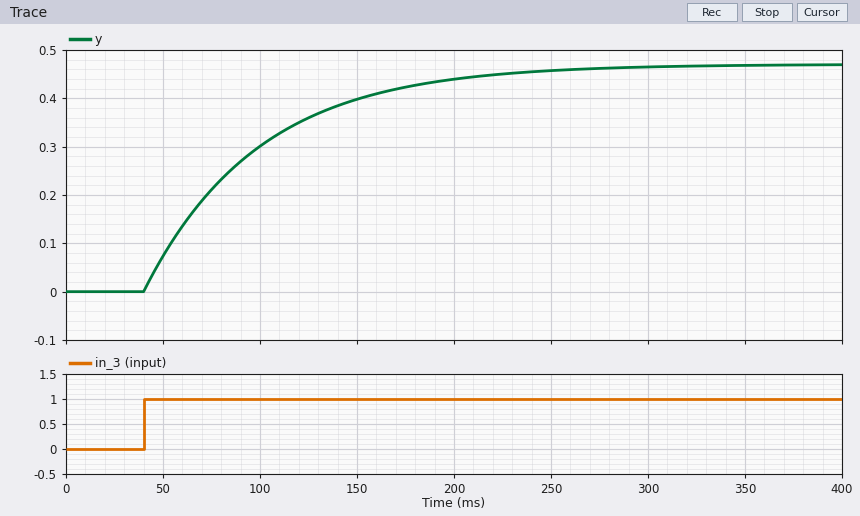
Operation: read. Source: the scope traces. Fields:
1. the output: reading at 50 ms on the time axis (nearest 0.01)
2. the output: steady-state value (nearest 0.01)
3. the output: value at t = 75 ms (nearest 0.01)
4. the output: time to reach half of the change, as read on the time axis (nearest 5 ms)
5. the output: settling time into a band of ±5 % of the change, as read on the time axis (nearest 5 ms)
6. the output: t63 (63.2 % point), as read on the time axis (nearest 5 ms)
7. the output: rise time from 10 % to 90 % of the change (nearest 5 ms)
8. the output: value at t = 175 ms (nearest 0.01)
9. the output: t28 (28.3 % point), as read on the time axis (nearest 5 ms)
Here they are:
0.07
0.47
0.21
80 ms
215 ms
100 ms
130 ms
0.42
60 ms
